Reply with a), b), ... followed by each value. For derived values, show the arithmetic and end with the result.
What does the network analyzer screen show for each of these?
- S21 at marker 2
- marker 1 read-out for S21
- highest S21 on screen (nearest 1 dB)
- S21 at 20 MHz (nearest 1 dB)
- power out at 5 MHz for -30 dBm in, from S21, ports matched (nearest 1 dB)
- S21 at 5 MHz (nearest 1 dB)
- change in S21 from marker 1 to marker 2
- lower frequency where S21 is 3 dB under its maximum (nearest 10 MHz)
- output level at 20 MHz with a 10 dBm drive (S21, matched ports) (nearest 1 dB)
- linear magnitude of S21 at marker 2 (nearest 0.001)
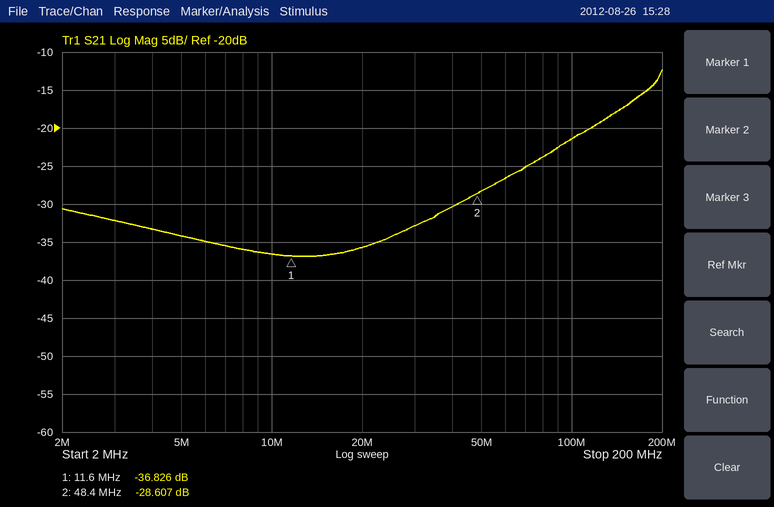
a) -28.607 dB
b) -36.826 dB
c) -12 dB
d) -36 dB
e) -30 dBm + (-34 dB) = -64 dBm
f) -34 dB
g) -28.607 − (-36.826) = 8.219 dB
h) 170 MHz
i) 10 dBm + (-36 dB) = -26 dBm
j) 10^(-28.607/20) ≈ 0.037
